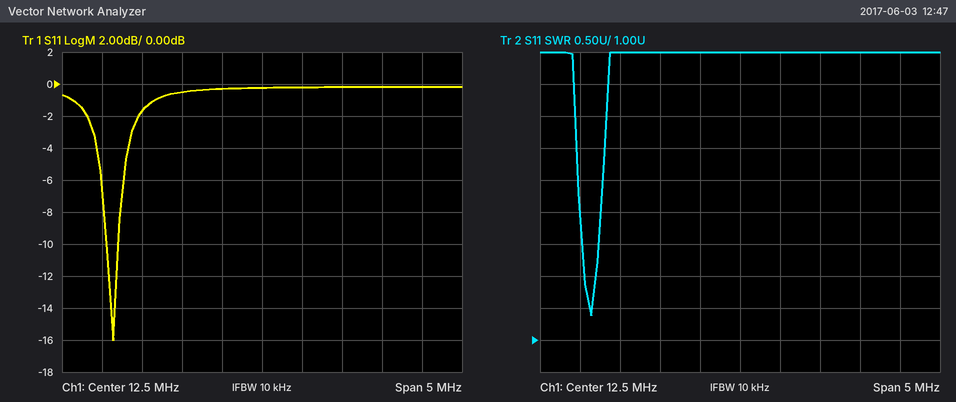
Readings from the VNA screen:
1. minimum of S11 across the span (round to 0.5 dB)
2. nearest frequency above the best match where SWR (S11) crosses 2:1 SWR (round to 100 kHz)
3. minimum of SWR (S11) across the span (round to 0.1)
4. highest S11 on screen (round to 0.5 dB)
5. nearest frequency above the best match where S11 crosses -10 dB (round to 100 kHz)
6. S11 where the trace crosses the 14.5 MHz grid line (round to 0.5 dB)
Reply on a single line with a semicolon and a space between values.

-16.0 dB; 10.7 MHz; 1.4; 0.0 dB; 10.7 MHz; 0.0 dB
